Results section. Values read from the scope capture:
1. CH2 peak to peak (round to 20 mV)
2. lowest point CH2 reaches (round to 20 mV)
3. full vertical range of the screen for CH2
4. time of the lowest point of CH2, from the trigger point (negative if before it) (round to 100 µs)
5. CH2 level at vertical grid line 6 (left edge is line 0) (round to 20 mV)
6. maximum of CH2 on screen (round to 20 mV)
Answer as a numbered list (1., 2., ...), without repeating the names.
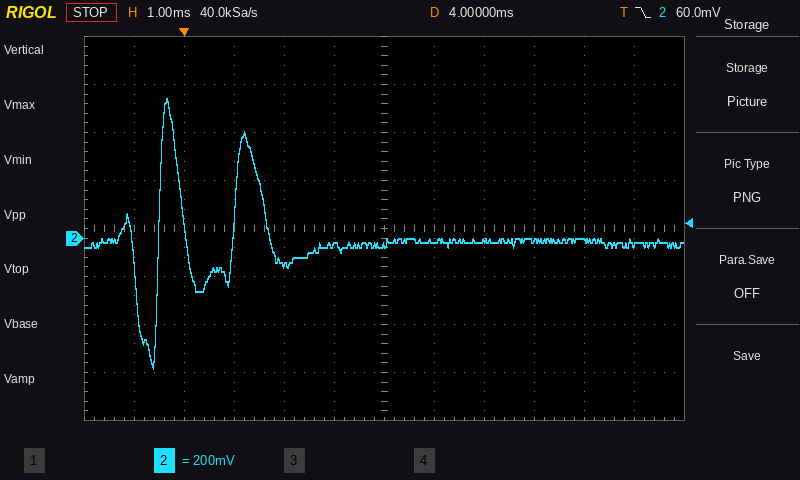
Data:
1. 1.12 V
2. -540 mV
3. 1.6 V
4. -600 µs
5. -20 mV
6. 580 mV
